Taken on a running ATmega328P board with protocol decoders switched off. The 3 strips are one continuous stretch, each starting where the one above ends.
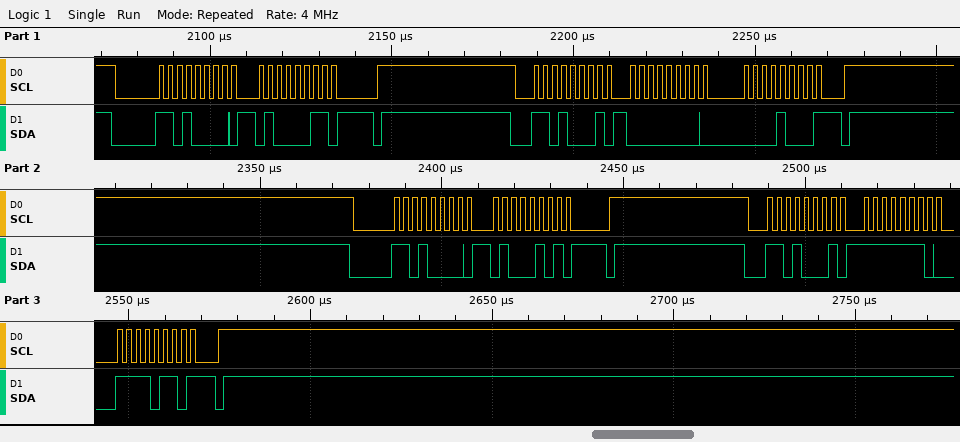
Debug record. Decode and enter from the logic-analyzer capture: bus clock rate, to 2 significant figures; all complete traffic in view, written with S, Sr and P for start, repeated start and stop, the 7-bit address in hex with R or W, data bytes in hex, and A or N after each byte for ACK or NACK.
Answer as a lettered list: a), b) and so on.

a) 400 kHz
b) S 68W A 43 A P S 68R A 00 A 08 N P S 68W A 45 A P S 68R A FE A F6 N P
